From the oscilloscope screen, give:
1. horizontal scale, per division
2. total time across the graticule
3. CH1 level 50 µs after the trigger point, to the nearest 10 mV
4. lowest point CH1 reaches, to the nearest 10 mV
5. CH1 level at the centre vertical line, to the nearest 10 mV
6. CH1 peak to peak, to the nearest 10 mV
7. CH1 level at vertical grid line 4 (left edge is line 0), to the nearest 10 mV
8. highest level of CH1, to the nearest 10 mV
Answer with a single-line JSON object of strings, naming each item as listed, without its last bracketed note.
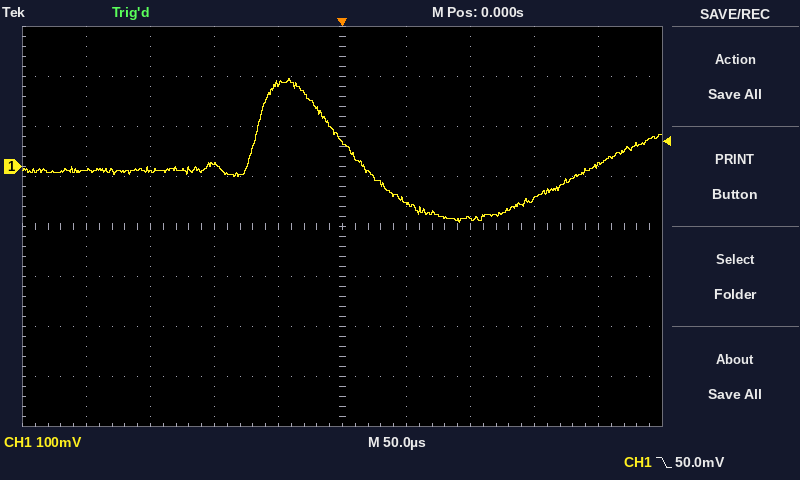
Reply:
{"horizontal scale, per division": "50 µs", "total time across the graticule": "500 µs", "CH1 level 50 µs after the trigger point, to the nearest 10 mV": "-70 mV", "lowest point CH1 reaches, to the nearest 10 mV": "-110 mV", "CH1 level at the centre vertical line, to the nearest 10 mV": "50 mV", "CH1 peak to peak, to the nearest 10 mV": "290 mV", "CH1 level at vertical grid line 4 (left edge is line 0), to the nearest 10 mV": "170 mV", "highest level of CH1, to the nearest 10 mV": "180 mV"}
